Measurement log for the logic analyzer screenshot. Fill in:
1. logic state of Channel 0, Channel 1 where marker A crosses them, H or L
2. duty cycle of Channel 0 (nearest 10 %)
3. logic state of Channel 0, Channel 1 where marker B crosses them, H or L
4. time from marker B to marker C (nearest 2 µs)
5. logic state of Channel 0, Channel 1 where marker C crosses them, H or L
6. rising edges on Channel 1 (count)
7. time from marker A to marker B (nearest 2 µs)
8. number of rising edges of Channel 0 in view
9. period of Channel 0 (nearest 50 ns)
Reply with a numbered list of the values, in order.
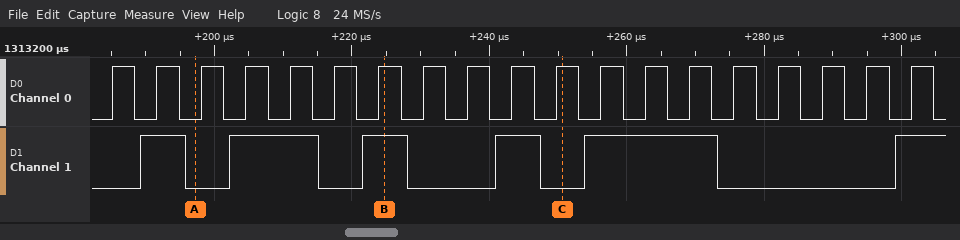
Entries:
1. Channel 0=L, Channel 1=L
2. 50 %
3. Channel 0=H, Channel 1=H
4. 26 µs
5. Channel 0=H, Channel 1=L
6. 6
7. 28 µs
8. 19
9. 6450 ns
